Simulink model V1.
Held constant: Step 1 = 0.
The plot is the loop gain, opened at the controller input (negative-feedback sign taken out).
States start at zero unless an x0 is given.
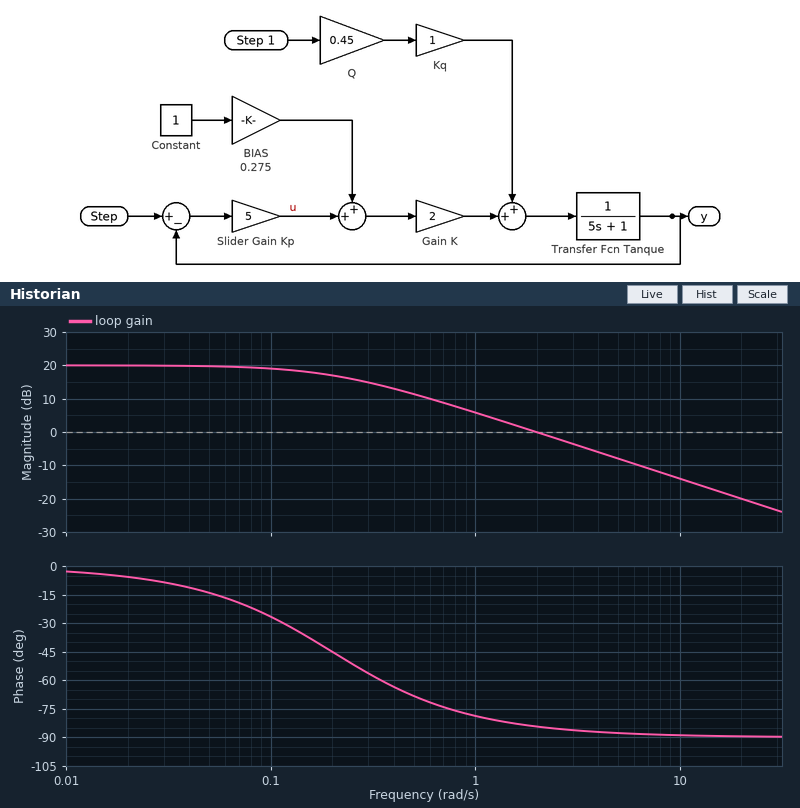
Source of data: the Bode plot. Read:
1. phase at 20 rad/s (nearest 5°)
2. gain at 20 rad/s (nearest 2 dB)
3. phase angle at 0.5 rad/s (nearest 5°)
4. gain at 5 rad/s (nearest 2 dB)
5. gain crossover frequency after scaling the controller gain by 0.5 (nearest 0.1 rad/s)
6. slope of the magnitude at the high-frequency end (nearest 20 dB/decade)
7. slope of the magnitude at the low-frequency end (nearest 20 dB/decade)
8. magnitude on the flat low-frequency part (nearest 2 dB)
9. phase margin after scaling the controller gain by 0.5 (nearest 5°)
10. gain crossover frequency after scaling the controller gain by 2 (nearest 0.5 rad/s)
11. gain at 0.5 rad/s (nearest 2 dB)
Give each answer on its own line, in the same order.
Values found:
-90°
-20 dB
-70°
-8 dB
1.0 rad/s
-20 dB/decade
0 dB/decade
20 dB
100°
4.0 rad/s
12 dB
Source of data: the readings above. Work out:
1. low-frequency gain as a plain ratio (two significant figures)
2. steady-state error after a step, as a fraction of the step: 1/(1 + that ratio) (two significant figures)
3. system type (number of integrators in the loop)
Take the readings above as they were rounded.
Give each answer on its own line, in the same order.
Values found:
10
0.091
0
